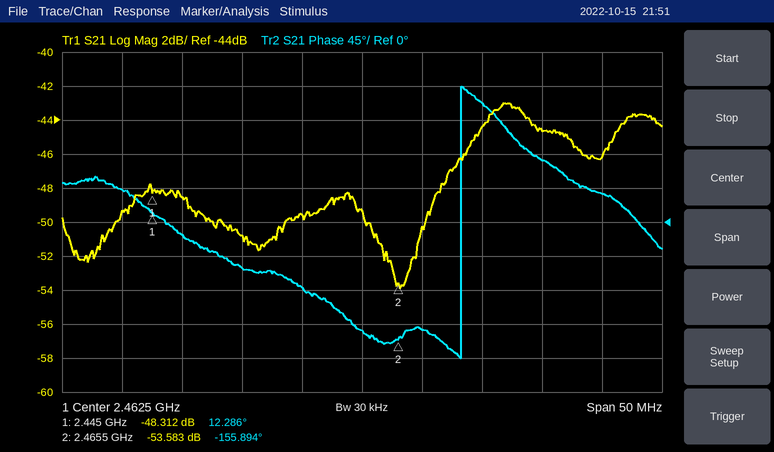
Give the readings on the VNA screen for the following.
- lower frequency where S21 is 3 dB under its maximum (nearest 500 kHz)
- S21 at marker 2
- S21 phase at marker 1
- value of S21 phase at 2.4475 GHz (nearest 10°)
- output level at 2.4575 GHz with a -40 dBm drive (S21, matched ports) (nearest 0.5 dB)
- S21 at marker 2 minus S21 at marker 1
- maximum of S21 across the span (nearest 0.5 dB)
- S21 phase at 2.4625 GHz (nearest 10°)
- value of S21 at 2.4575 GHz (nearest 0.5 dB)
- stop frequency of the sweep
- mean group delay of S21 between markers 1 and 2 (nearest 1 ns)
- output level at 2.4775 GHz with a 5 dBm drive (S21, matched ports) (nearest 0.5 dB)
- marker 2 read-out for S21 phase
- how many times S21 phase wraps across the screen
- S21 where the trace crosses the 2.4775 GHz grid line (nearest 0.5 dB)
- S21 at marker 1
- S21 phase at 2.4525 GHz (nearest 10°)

2.4710 GHz
-53.583 dB
12.286°
-20°
-89.5 dBm
-5.271 dB
-43.0 dB
-140°
-49.5 dB
2.4875 GHz
23 ns
-39.5 dBm
-155.894°
1
-44.5 dB
-48.312 dB
-60°
